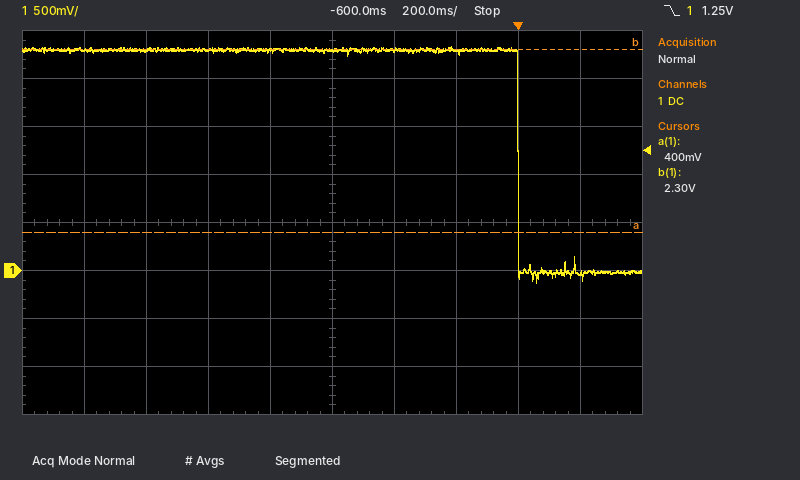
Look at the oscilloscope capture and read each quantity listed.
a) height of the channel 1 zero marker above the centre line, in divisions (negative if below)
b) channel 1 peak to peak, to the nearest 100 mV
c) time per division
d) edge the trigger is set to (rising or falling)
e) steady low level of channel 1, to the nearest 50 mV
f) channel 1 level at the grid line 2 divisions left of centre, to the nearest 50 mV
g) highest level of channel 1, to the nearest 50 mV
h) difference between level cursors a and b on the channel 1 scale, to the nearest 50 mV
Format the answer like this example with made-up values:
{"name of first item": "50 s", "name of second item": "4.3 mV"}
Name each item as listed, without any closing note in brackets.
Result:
{"height of the channel 1 zero marker above the centre line, in divisions": "-1.0 div", "channel 1 peak to peak, to the nearest 100 mV": "2.50 V", "time per division": "200 ms", "edge the trigger is set to": "falling", "steady low level of channel 1, to the nearest 50 mV": "0 mV", "channel 1 level at the grid line 2 divisions left of centre, to the nearest 50 mV": "2.30 V", "highest level of channel 1, to the nearest 50 mV": "2.35 V", "difference between level cursors a and b on the channel 1 scale, to the nearest 50 mV": "1.90 V"}
